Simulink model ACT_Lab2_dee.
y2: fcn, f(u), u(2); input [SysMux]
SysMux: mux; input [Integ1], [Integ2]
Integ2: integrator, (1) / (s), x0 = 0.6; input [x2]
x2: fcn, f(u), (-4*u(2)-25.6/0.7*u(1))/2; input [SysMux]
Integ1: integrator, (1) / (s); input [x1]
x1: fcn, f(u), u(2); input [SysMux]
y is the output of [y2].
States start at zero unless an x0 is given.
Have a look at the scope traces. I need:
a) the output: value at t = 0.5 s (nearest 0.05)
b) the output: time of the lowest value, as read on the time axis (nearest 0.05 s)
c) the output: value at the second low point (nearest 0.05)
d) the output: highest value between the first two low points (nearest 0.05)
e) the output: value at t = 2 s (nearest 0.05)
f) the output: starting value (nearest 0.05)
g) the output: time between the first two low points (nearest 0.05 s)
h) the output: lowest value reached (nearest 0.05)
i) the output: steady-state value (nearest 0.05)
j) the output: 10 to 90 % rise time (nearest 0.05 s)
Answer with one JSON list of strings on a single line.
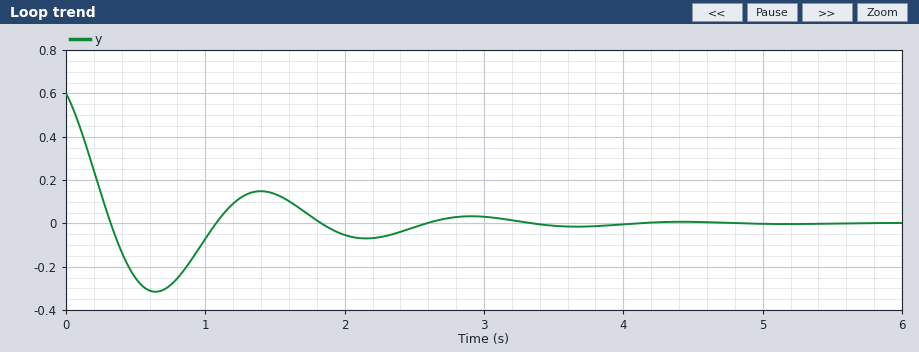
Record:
["-0.25", "0.65 s", "-0.05", "0.15", "-0.05", "0.60", "1.50 s", "-0.30", "0.00", "0.25 s"]
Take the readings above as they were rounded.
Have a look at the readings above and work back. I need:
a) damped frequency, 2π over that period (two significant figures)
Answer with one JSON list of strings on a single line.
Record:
["4.2 rad/s"]
